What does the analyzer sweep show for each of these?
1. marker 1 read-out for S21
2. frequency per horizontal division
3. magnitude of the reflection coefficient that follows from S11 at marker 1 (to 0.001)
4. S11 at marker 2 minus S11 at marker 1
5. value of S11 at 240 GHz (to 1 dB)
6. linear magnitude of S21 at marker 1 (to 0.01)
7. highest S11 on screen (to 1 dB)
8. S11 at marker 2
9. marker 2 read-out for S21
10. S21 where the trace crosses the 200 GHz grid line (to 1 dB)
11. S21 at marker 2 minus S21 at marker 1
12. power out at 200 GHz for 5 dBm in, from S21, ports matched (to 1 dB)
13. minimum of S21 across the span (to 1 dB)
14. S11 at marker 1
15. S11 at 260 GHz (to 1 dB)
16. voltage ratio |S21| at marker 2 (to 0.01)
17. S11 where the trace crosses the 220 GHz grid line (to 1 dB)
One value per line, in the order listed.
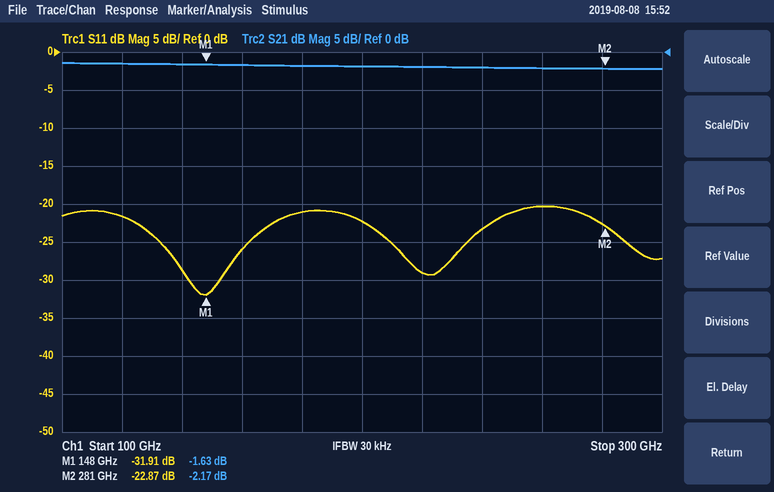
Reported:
-1.63 dB
20 GHz
0.025
9.04 dB
-23 dB
0.83
-20 dB
-22.87 dB
-2.17 dB
-2 dB
-0.54 dB
3 dBm
-2 dB
-31.91 dB
-20 dB
0.78
-29 dB
